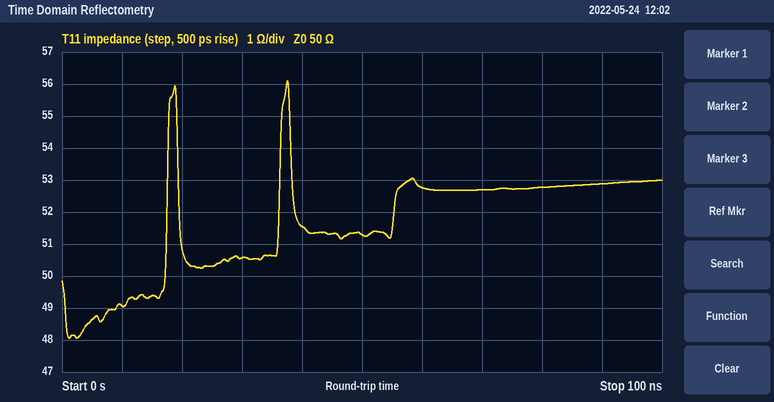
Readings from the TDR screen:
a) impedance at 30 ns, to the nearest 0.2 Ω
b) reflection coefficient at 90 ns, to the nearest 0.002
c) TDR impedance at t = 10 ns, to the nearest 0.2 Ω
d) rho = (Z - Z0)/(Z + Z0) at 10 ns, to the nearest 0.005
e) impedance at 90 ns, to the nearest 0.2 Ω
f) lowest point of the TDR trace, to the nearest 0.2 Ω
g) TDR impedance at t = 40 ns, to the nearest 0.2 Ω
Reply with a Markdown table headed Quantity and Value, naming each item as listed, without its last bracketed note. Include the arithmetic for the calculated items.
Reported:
| Quantity | Value |
|---|---|
| impedance at 30 ns, to the nearest 0.2 Ω | 50.6 Ω |
| reflection coefficient at 90 ns, to the nearest 0.002 | (52.8 − 50)/(52.8 + 50) ≈ +0.0272, so +0.028 to the nearest 0.002 |
| TDR impedance at t = 10 ns, to the nearest 0.2 Ω | 49.0 Ω |
| rho = (Z - Z0)/(Z + Z0) at 10 ns, to the nearest 0.005 | (49 − 50)/(49 + 50) ≈ -0.010 |
| impedance at 90 ns, to the nearest 0.2 Ω | 52.8 Ω |
| lowest point of the TDR trace, to the nearest 0.2 Ω | 48.0 Ω |
| TDR impedance at t = 40 ns, to the nearest 0.2 Ω | 51.6 Ω |
